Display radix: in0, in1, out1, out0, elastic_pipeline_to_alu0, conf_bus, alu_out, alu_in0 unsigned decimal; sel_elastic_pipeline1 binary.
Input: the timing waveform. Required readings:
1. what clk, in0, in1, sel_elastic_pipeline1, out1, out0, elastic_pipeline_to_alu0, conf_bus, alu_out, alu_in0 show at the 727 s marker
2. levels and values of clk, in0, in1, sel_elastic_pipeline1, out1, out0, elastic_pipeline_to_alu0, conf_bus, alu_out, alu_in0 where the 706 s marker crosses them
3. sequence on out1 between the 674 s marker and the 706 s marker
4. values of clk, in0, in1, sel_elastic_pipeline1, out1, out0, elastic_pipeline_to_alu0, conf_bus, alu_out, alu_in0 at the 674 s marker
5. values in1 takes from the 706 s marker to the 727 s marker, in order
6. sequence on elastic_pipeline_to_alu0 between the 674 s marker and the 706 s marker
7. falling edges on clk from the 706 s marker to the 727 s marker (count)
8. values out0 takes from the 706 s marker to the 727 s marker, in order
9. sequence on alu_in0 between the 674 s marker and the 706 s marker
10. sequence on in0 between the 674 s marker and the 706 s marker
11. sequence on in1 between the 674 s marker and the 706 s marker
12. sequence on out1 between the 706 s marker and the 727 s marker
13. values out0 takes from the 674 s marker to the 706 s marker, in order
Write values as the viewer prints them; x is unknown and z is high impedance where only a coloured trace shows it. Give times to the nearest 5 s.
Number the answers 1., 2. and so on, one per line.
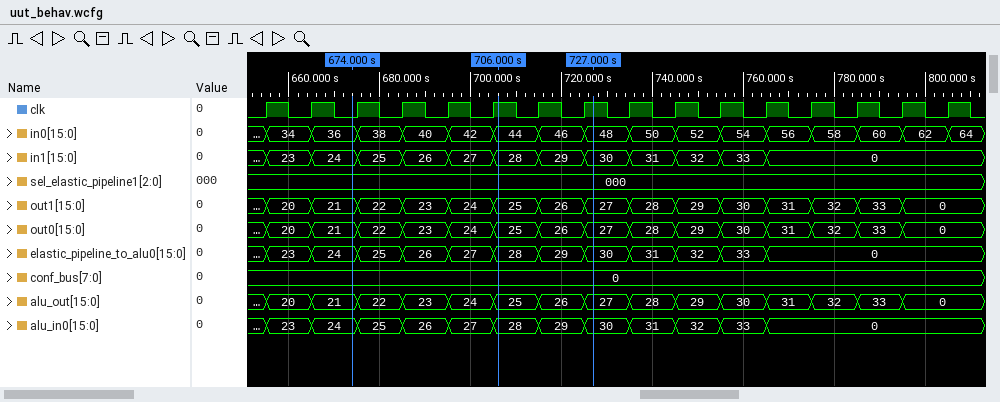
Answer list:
1. clk=1, in0=48, in1=30, sel_elastic_pipeline1=000, out1=27, out0=27, elastic_pipeline_to_alu0=30, conf_bus=0, alu_out=27, alu_in0=30
2. clk=1, in0=44, in1=28, sel_elastic_pipeline1=000, out1=25, out0=25, elastic_pipeline_to_alu0=28, conf_bus=0, alu_out=25, alu_in0=28
3. 21, 22, 23, 24, 25
4. clk=0, in0=36, in1=24, sel_elastic_pipeline1=000, out1=21, out0=21, elastic_pipeline_to_alu0=24, conf_bus=0, alu_out=21, alu_in0=24
5. 28, 29, 30
6. 24, 25, 26, 27, 28
7. 2
8. 25, 26, 27
9. 24, 25, 26, 27, 28
10. 36, 38, 40, 42, 44
11. 24, 25, 26, 27, 28
12. 25, 26, 27
13. 21, 22, 23, 24, 25
